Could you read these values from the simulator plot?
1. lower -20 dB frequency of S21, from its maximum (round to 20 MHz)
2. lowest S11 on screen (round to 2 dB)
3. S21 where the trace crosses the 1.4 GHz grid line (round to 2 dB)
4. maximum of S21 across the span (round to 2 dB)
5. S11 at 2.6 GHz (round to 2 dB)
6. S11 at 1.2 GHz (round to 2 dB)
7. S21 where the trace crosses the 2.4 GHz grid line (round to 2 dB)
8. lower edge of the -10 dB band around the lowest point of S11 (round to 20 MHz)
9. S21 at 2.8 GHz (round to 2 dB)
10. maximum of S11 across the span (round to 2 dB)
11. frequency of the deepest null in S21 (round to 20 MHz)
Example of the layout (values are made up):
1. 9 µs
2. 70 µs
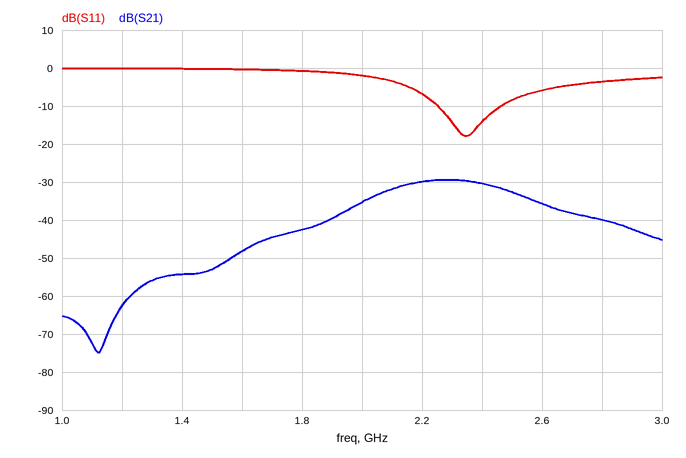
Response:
1. 1.58 GHz
2. -18 dB
3. -54 dB
4. -30 dB
5. -6 dB
6. 0 dB
7. -30 dB
8. 2.26 GHz
9. -40 dB
10. 0 dB
11. 1.12 GHz
